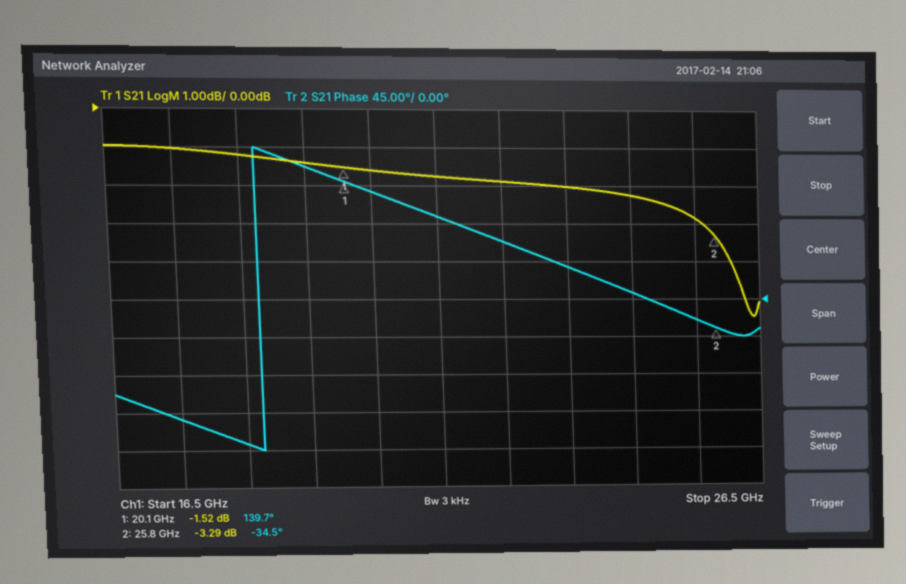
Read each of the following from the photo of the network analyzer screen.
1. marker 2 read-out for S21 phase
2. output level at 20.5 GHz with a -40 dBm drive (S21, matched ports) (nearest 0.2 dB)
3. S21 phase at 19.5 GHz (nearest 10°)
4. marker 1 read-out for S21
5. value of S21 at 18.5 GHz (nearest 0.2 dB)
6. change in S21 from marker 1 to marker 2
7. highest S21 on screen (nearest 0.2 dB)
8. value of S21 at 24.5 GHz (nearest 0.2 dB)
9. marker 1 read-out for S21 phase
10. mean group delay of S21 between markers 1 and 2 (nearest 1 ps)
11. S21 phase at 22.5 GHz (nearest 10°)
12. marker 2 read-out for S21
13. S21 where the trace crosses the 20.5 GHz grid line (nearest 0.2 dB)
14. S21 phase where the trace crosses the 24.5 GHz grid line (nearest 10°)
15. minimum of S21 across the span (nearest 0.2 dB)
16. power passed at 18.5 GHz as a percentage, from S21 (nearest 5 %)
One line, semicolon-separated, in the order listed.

-34.5°; -41.6 dBm; 160°; -1.52 dB; -1.2 dB; -1.77 dB; -1.0 dB; -2.2 dB; 139.7°; 85 ps; 70°; -3.29 dB; -1.6 dB; 10°; -5.4 dB; 75 %
